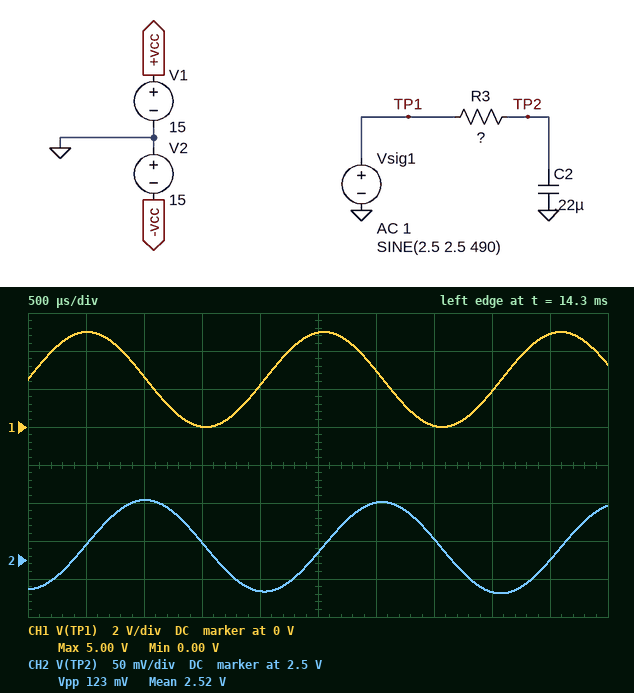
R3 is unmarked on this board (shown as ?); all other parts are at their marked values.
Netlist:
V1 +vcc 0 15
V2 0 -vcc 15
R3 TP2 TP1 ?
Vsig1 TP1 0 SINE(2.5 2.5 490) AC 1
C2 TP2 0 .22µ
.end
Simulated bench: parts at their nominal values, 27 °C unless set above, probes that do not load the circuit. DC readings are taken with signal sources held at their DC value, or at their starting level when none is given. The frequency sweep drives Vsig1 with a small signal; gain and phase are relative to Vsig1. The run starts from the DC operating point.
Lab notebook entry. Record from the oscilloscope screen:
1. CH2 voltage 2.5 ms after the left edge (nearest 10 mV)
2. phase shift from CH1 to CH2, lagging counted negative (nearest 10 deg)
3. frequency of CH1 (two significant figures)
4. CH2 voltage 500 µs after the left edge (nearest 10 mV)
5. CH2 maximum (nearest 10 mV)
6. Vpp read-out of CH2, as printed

2.51 V
-90 deg
490 Hz
2.52 V
2.58 V
123 mV
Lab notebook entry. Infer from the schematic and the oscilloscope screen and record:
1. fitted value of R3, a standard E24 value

62 kΩ
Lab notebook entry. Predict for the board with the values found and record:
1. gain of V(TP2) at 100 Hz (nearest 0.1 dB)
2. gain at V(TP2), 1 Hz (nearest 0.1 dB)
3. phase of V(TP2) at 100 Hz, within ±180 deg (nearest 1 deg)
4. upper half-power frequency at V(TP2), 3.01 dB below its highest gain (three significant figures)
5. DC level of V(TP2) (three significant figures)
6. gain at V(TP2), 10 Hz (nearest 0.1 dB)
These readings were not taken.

-18.7 dB
0 dB
-83 deg
11.7 Hz
2.50 V
-2.4 dB
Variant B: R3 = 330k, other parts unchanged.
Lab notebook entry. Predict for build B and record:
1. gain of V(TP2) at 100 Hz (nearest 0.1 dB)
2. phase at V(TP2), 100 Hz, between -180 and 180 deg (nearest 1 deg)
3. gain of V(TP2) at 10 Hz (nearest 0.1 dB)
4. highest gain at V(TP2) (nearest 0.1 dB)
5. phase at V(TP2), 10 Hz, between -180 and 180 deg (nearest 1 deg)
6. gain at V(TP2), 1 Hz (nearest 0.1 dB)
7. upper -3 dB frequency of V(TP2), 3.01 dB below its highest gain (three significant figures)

-33.2 dB
-89 deg
-13.4 dB
0 dB
-78 deg
-0.8 dB
2.19 Hz
